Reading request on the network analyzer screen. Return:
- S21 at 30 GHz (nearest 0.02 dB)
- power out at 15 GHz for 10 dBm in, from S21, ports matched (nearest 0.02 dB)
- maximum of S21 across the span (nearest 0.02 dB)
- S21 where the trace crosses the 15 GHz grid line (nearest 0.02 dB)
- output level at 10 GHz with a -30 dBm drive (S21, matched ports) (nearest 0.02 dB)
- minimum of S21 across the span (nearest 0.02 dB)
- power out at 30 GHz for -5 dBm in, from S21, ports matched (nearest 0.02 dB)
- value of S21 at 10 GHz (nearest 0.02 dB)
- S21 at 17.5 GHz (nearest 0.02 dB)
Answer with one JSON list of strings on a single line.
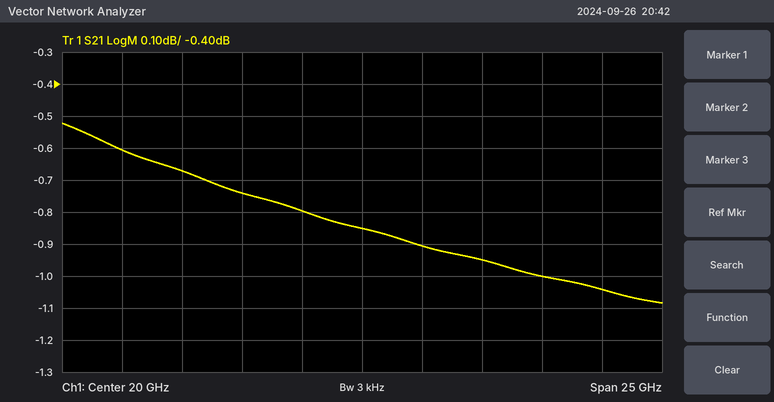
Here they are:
["-1.04 dB", "9.26 dBm", "-0.52 dB", "-0.74 dB", "-30.60 dBm", "-1.08 dB", "-6.04 dBm", "-0.60 dB", "-0.80 dB"]
